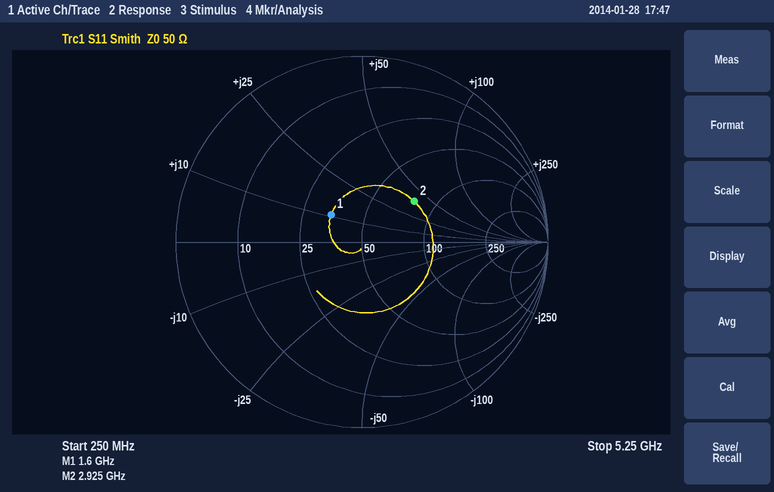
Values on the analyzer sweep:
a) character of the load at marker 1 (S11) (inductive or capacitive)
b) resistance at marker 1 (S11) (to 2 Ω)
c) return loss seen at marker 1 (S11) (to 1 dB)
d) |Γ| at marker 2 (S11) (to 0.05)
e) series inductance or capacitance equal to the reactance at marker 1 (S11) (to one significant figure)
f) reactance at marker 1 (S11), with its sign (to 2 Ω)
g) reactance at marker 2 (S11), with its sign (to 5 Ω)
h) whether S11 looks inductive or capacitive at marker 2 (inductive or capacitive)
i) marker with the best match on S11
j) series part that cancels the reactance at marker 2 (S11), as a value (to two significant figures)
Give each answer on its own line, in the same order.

inductive
34 Ω
13 dB
0.35
1 nH
+10 Ω
+40 Ω
inductive
marker 1
1.4 pF
